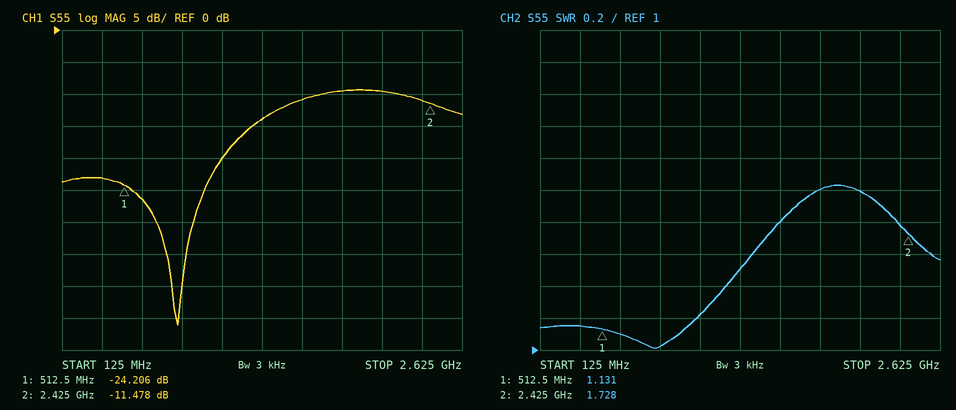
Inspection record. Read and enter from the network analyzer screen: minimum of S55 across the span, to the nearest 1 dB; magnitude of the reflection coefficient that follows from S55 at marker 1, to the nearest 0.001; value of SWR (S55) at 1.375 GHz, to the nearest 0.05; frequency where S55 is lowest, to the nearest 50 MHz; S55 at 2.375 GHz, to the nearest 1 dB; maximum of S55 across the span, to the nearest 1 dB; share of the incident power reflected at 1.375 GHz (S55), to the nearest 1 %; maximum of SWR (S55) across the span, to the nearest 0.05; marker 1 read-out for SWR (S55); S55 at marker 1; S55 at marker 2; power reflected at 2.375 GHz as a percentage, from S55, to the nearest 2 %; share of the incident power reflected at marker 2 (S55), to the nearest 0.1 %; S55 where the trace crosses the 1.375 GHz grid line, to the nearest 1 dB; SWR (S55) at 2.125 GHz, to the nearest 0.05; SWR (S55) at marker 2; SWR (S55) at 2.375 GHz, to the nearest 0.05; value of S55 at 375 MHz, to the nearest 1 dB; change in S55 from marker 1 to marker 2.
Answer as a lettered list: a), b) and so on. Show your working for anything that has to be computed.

a) -46 dB
b) 10^(-24.206/20) ≈ 0.062
c) 1.50
d) 850 MHz
e) -11 dB
f) -9 dB
g) 10^(-14/10) ≈ 4 %
h) 2.05
i) 1.131
j) -24.206 dB
k) -11.478 dB
l) 10^(-11/10) ≈ 8 %
m) 10^(-11.478/10) ≈ 7.1 %
n) -14 dB
o) 2.00
p) 1.728
q) 1.80
r) -23 dB
s) -11.478 − (-24.206) = 12.728 dB
